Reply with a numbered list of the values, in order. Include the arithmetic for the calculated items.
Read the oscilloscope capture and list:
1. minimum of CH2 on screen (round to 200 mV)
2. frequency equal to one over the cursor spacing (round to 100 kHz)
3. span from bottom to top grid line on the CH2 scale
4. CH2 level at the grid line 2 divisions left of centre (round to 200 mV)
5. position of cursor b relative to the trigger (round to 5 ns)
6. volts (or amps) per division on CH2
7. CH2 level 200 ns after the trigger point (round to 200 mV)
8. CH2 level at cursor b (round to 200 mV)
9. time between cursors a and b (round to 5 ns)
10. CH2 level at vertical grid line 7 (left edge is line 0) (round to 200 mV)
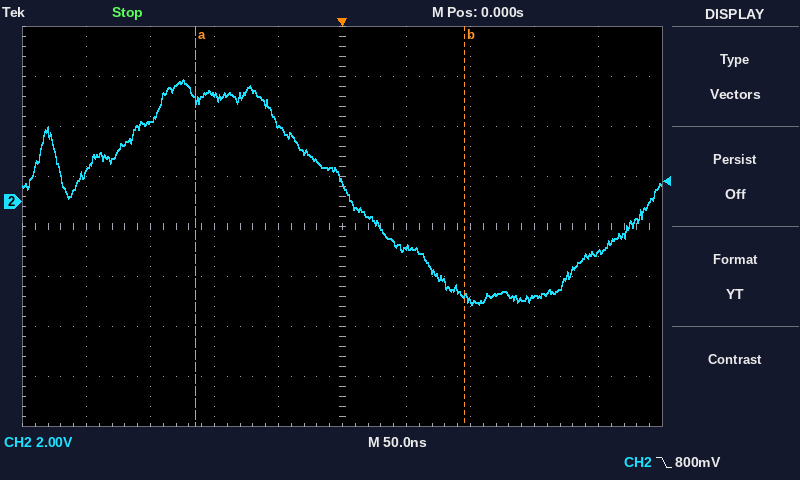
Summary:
1. -4.2 V
2. 1 / 210 ns ≈ 4.8 MHz
3. 16 V
4. 4.2 V
5. +95 ns
6. 2 V
7. -2.0 V
8. -3.8 V
9. 210 ns
10. -4.0 V
